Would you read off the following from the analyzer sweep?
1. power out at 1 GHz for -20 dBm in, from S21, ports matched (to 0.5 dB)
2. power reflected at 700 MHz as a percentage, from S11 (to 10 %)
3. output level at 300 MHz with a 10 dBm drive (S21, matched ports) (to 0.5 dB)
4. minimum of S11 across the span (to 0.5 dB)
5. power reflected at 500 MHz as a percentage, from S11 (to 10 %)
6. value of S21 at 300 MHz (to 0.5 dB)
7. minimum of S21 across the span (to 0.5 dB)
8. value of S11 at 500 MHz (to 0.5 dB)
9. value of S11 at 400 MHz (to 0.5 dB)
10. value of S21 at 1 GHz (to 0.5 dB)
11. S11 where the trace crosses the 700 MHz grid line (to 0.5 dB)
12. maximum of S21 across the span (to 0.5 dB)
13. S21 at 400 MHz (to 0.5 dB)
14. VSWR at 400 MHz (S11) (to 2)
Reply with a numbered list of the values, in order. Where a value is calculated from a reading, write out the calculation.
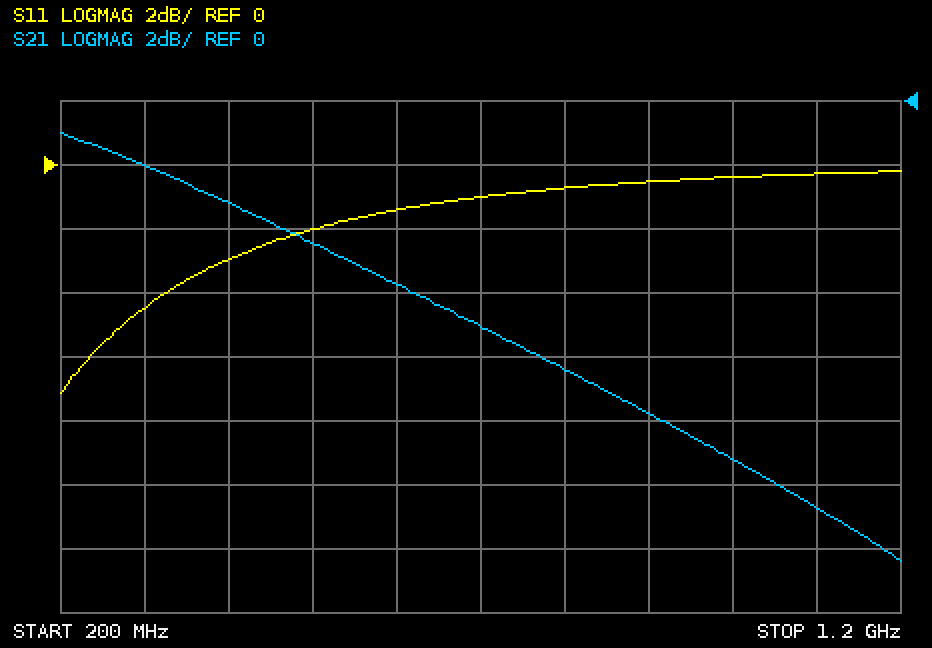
1. -20 dBm + (-11.0 dB) = -31.0 dBm
2. 10^(-1/10) ≈ 79.4 %, so 80 % to the nearest 10 %
3. 10 dBm + (-2.0 dB) = 8.0 dBm
4. -7.0 dB
5. 10^(-2/10) ≈ 63.1 %, so 60 % to the nearest 10 %
6. -2.0 dB
7. -14.5 dB
8. -2.0 dB
9. -3.0 dB
10. -11.0 dB
11. -1.0 dB
12. -1.0 dB
13. -3.0 dB
14. |Γ| = 10^(-3/20) = 0.7079; VSWR = (1 + 0.7079)/(1 − 0.7079) ≈ 6
